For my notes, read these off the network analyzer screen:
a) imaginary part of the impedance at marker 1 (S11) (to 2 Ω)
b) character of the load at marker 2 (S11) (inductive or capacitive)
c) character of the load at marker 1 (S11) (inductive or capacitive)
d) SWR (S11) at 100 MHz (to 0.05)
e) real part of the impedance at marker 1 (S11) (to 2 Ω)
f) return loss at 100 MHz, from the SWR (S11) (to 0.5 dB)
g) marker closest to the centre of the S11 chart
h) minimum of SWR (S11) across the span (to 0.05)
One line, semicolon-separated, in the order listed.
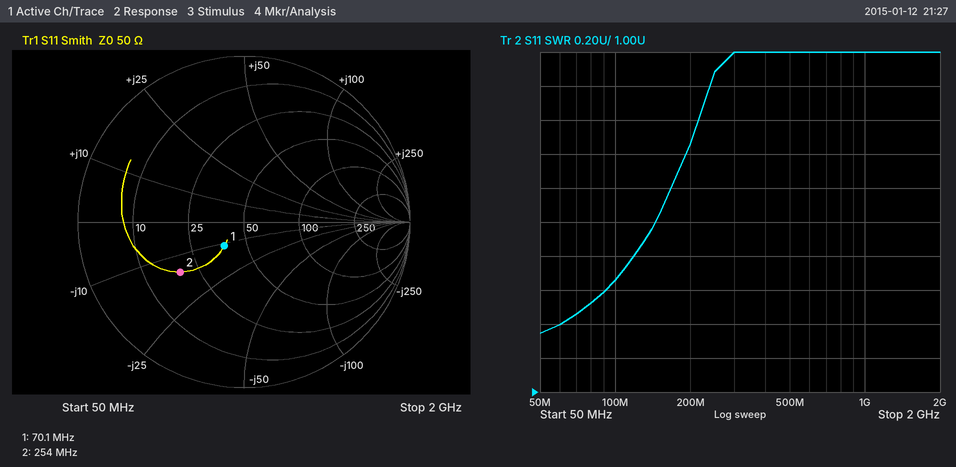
-12 Ω; capacitive; capacitive; 1.65; 38 Ω; 12.0 dB; marker 1; 1.35
